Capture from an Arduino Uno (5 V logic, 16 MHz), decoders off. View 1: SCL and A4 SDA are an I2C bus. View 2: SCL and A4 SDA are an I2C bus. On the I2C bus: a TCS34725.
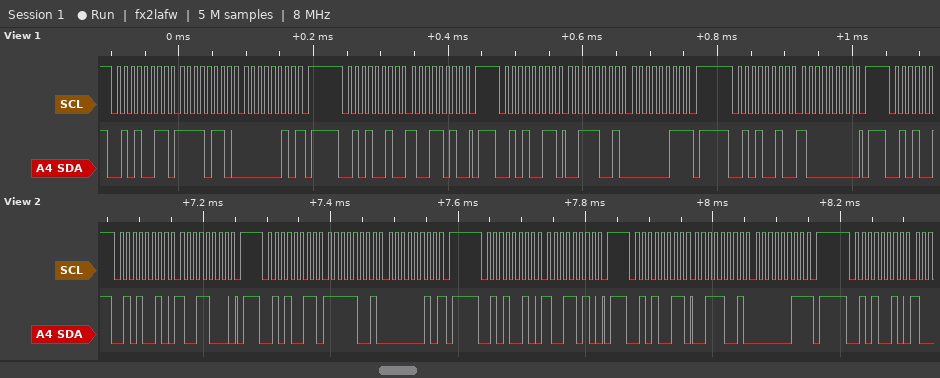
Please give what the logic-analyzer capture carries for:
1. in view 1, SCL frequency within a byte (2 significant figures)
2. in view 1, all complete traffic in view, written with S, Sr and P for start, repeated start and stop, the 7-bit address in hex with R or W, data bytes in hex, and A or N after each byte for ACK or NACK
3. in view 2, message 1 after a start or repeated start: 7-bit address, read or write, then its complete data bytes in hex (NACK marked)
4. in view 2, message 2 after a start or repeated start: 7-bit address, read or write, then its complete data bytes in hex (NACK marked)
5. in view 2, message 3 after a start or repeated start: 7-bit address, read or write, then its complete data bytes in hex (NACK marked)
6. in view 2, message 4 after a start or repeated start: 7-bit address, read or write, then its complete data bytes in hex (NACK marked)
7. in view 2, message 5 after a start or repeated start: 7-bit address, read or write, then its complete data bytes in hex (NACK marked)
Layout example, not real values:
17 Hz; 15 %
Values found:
100 kHz; S 29R A F6 A 02 N P S 29W A 9A A P S 29R A 39 A 03 N P S 29W A 80 A P; 0x29 write: 98; 0x29 read: F9 02 NACK; 0x29 write: 9A; 0x29 read: 39 03 NACK; 0x29 write
